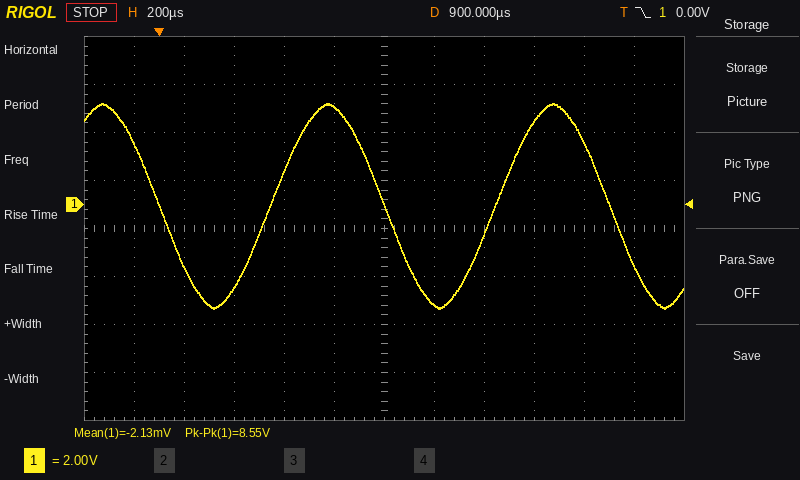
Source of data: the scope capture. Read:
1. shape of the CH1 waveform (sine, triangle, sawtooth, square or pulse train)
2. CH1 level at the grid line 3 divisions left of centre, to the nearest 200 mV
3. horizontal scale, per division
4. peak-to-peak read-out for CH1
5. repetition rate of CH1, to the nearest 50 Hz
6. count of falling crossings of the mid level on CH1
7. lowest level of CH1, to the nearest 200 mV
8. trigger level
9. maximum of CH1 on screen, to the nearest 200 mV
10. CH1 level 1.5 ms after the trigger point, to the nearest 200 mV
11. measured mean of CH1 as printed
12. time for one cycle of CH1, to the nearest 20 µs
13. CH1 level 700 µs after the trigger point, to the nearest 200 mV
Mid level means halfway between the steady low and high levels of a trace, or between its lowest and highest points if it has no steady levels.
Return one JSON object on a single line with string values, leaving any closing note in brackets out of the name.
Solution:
{"shape of the CH1 waveform": "sine", "CH1 level at the grid line 3 divisions left of centre, to the nearest 200 mV": "-3.4 V", "horizontal scale, per division": "200 µs", "peak-to-peak read-out for CH1": "8.55 V", "repetition rate of CH1, to the nearest 50 Hz": "1.10 kHz", "count of falling crossings of the mid level on CH1": "3", "lowest level of CH1, to the nearest 200 mV": "-4.4 V", "trigger level": "0.00 V", "maximum of CH1 on screen, to the nearest 200 mV": "4.2 V", "CH1 level 1.5 ms after the trigger point, to the nearest 200 mV": "3.4 V", "measured mean of CH1 as printed": "-2.13 mV", "time for one cycle of CH1, to the nearest 20 µs": "900 µs", "CH1 level 700 µs after the trigger point, to the nearest 200 mV": "4.0 V"}
